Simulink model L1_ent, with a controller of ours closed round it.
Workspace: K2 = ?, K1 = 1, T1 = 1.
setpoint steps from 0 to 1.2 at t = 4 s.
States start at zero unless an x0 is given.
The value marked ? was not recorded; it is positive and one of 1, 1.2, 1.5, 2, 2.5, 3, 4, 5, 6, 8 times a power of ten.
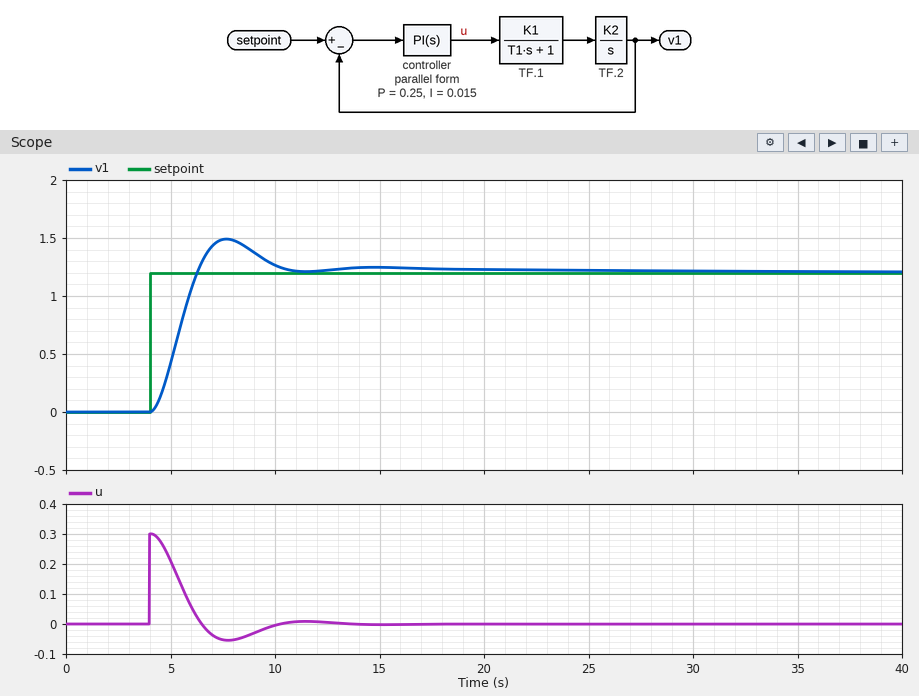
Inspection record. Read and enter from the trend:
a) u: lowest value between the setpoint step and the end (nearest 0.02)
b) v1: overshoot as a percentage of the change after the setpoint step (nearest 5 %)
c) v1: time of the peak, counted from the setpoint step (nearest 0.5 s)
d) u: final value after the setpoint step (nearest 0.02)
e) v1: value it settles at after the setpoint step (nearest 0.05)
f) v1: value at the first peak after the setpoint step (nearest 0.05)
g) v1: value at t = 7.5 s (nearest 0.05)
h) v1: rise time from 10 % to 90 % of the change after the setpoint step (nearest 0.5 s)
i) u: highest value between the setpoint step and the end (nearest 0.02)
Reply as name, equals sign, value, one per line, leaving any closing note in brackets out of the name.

u: lowest value between the setpoint step and the end = -0.06
v1: overshoot as a percentage of the change after the setpoint step = 25 %
v1: time of the peak, counted from the setpoint step = 3.5 s
u: final value after the setpoint step = 0.00
v1: value it settles at after the setpoint step = 1.20
v1: value at the first peak after the setpoint step = 1.50
v1: value at t = 7.5 s = 1.50
v1: rise time from 10 % to 90 % of the change after the setpoint step = 1.5 s
u: highest value between the setpoint step and the end = 0.30
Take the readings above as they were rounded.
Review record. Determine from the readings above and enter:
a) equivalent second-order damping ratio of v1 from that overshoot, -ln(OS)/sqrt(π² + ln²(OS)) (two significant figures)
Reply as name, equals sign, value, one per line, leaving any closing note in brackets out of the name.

equivalent second-order damping ratio of v1 from that overshoot, -ln(OS)/sqrt(π² + ln²(OS)) = 0.40
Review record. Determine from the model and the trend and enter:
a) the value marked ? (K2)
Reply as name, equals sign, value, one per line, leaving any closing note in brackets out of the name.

the value marked ? = 4
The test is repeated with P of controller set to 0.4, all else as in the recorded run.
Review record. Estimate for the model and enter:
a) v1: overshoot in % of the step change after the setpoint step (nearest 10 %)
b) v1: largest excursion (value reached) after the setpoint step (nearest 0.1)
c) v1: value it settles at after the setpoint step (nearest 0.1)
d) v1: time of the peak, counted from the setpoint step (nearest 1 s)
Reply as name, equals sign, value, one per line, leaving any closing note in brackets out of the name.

v1: overshoot in % of the step change after the setpoint step = 30 %
v1: largest excursion (value reached) after the setpoint step = 1.6
v1: value it settles at after the setpoint step = 1.2
v1: time of the peak, counted from the setpoint step = 3 s
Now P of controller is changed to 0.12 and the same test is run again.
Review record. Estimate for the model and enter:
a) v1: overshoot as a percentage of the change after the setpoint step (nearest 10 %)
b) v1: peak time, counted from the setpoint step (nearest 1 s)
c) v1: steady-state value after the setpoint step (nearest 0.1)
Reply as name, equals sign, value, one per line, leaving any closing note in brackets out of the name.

v1: overshoot as a percentage of the change after the setpoint step = 30 %
v1: peak time, counted from the setpoint step = 6 s
v1: steady-state value after the setpoint step = 1.2
